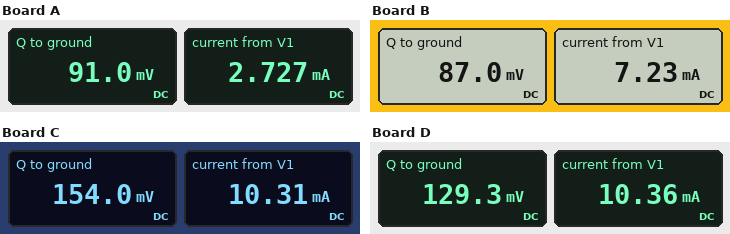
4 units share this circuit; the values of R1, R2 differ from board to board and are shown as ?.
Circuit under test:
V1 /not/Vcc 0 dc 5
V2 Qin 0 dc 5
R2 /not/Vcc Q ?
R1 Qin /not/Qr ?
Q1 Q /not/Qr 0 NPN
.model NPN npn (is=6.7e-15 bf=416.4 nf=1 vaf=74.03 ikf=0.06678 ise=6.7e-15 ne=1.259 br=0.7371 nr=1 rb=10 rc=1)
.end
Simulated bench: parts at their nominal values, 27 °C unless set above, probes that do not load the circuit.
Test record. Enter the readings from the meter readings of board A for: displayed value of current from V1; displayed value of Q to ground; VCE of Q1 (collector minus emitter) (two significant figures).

2.727 mA
91.0 mV
91 mV
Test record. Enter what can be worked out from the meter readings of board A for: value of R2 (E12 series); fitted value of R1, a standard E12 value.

1.8 kΩ
27 kΩ
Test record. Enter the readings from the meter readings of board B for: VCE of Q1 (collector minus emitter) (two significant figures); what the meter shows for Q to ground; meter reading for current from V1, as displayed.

87 mV
87.0 mV
7.23 mA
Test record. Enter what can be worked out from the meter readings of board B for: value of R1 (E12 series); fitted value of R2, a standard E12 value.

6.8 kΩ
680 Ω
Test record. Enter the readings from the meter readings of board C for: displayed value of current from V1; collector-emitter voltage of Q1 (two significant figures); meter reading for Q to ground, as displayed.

10.31 mA
150 mV
154.0 mV
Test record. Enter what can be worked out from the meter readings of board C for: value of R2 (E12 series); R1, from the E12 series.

470 Ω
33 kΩ
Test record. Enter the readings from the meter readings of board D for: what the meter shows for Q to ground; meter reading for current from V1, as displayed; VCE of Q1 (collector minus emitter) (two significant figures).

129.3 mV
10.36 mA
130 mV
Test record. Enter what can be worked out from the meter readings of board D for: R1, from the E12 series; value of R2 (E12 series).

18 kΩ
470 Ω
